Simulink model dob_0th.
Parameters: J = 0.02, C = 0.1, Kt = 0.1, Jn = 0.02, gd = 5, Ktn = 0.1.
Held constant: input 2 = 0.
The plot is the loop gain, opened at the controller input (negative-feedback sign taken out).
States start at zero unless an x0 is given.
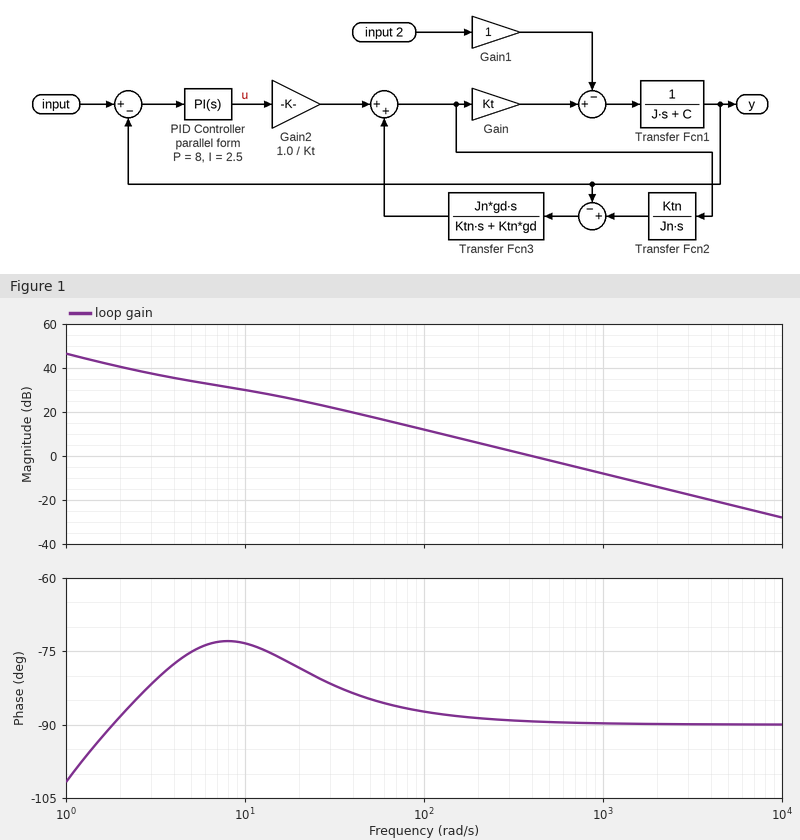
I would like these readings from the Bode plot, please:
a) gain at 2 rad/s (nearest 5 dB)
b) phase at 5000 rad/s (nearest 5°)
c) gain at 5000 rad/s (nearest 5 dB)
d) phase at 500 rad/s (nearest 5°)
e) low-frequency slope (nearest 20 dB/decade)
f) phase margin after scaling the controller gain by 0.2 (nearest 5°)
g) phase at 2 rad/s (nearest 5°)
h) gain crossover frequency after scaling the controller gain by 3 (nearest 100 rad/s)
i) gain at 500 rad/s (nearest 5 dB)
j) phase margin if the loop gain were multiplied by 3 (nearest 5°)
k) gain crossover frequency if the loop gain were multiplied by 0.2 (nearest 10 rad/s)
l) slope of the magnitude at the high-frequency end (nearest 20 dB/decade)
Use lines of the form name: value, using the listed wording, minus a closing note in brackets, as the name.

gain at 2 rad/s: 40 dB
phase at 5000 rad/s: -90°
gain at 5000 rad/s: -20 dB
phase at 500 rad/s: -90°
low-frequency slope: -20 dB/decade
phase margin after scaling the controller gain by 0.2: 95°
phase at 2 rad/s: -90°
gain crossover frequency after scaling the controller gain by 3: 1200 rad/s
gain at 500 rad/s: 0 dB
phase margin if the loop gain were multiplied by 3: 90°
gain crossover frequency if the loop gain were multiplied by 0.2: 80 rad/s
slope of the magnitude at the high-frequency end: -20 dB/decade
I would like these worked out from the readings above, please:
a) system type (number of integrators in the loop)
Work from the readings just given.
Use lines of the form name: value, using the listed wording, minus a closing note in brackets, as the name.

system type: 1
